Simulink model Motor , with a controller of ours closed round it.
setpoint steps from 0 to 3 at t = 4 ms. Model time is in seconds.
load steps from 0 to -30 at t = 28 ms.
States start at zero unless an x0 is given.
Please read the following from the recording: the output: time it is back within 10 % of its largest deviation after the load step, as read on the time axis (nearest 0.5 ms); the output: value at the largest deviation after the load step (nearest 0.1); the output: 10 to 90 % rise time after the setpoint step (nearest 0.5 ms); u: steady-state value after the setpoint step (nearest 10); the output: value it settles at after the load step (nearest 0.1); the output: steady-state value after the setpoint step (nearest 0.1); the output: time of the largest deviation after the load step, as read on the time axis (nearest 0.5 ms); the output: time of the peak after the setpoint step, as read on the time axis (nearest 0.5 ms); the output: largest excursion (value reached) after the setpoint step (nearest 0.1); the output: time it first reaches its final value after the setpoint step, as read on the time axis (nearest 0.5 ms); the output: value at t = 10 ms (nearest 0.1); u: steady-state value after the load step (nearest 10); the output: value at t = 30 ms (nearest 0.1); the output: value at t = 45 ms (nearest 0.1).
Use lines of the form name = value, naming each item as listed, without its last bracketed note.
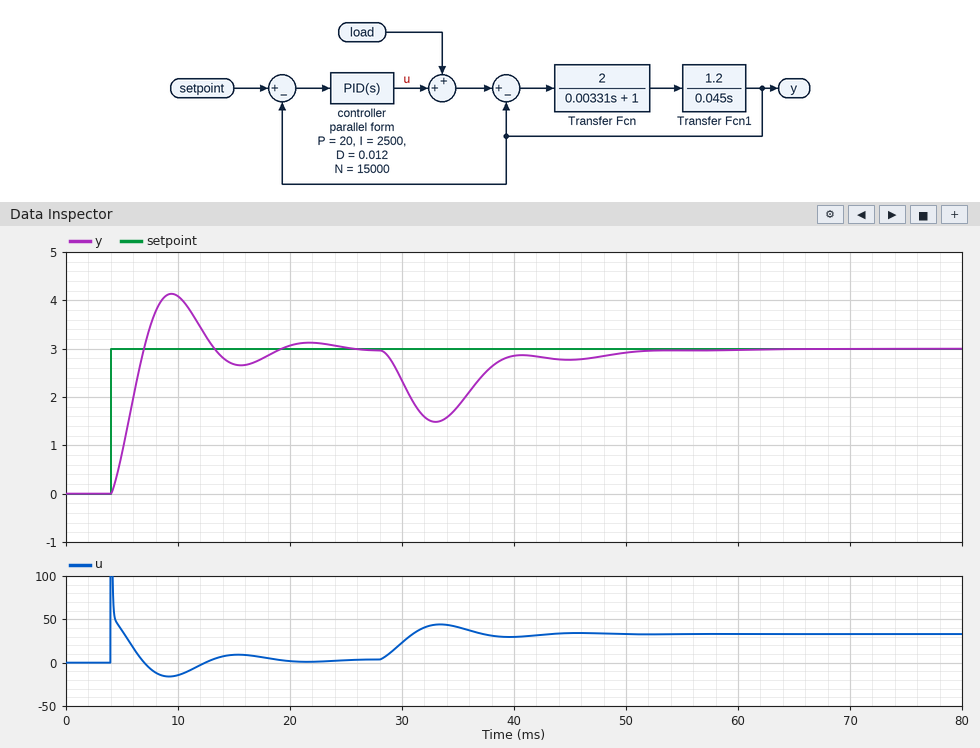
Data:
the output: time it is back within 10 % of its largest deviation after the load step, as read on the time axis = 48.0 ms
the output: value at the largest deviation after the load step = 1.5
the output: 10 to 90 % rise time after the setpoint step = 2.0 ms
u: steady-state value after the setpoint step = 0
the output: value it settles at after the load step = 3.0
the output: steady-state value after the setpoint step = 3.0
the output: time of the largest deviation after the load step, as read on the time axis = 33.0 ms
the output: time of the peak after the setpoint step, as read on the time axis = 9.5 ms
the output: largest excursion (value reached) after the setpoint step = 4.1
the output: time it first reaches its final value after the setpoint step, as read on the time axis = 7.0 ms
the output: value at t = 10 ms = 4.1
u: steady-state value after the load step = 30
the output: value at t = 30 ms = 2.3
the output: value at t = 45 ms = 2.8
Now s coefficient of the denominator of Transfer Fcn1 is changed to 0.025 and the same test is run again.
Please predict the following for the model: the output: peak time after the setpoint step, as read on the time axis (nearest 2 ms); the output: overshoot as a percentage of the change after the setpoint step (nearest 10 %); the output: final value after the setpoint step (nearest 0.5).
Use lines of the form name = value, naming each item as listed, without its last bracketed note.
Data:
the output: peak time after the setpoint step, as read on the time axis = 8 ms
the output: overshoot as a percentage of the change after the setpoint step = 30 %
the output: final value after the setpoint step = 3.0
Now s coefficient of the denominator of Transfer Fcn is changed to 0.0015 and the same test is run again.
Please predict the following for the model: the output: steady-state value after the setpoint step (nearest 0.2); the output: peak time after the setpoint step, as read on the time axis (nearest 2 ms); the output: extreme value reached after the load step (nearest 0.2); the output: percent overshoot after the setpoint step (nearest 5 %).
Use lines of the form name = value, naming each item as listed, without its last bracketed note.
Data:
the output: steady-state value after the setpoint step = 3.0
the output: peak time after the setpoint step, as read on the time axis = 8 ms
the output: extreme value reached after the load step = 1.6
the output: percent overshoot after the setpoint step = 15 %
